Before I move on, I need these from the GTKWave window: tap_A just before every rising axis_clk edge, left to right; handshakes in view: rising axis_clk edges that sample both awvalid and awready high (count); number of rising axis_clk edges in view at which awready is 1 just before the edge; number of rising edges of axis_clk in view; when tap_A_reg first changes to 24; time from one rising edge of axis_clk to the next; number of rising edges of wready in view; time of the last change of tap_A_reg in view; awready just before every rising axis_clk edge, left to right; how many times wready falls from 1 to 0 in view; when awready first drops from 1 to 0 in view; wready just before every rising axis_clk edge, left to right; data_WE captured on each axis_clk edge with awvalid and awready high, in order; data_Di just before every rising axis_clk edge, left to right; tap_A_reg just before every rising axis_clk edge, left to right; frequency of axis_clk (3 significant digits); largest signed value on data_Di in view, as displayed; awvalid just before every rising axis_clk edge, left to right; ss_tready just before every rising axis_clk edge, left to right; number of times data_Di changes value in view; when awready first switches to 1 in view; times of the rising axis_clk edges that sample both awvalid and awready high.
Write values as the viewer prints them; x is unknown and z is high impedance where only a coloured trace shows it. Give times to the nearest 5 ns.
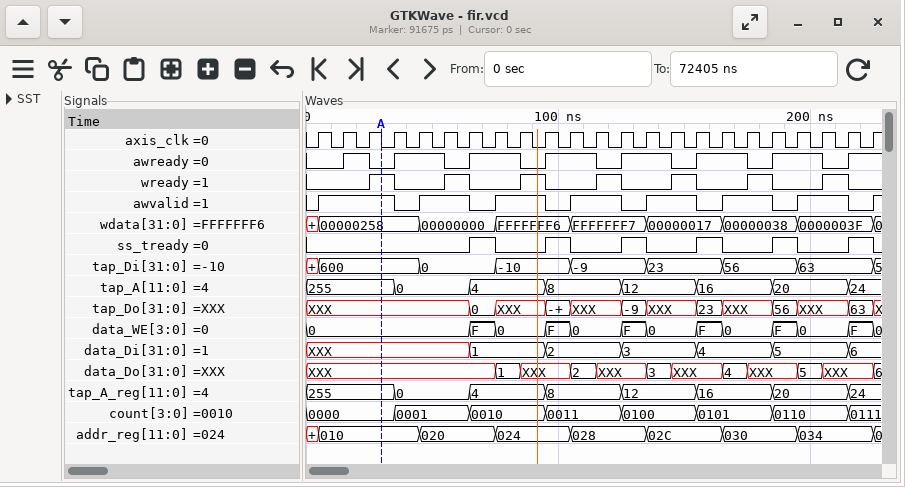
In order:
255, 255, 255, 255, 0, 0, 0, 4, 4, 4, 8, 8, 8, 12, 12, 12, 16, 16, 16, 20, 20, 20, 24
7
14
23
215 ns
10 ns
7
215 ns
0 0 1 0 1 1 0 1 1 0 1 1 0 1 1 0 1 1 0 1 1 0 1
7
25 ns
0 0 0 1 0 0 1 0 0 1 0 0 1 0 0 1 0 0 1 0 0 1 0
0, 0, 0, 0, 0, 0, 0
XXX, XXX, XXX, XXX, XXX, XXX, XXX, 1, 1, 1, 2, 2, 2, 3, 3, 3, 4, 4, 4, 5, 5, 5, 6
255, 255, 255, 255, 0, 0, 0, 4, 4, 4, 8, 8, 8, 12, 12, 12, 16, 16, 16, 20, 20, 20, 24
100 MHz
6
0 1 1 1 0 1 1 0 1 1 0 1 1 0 1 1 0 1 1 0 1 1 0
0 0 0 0 0 0 0 1 0 0 1 0 0 1 0 0 1 0 0 1 0 0 1
6
15 ns
25 ns, 55 ns, 85 ns, 115 ns, 145 ns, 175 ns, 205 ns
